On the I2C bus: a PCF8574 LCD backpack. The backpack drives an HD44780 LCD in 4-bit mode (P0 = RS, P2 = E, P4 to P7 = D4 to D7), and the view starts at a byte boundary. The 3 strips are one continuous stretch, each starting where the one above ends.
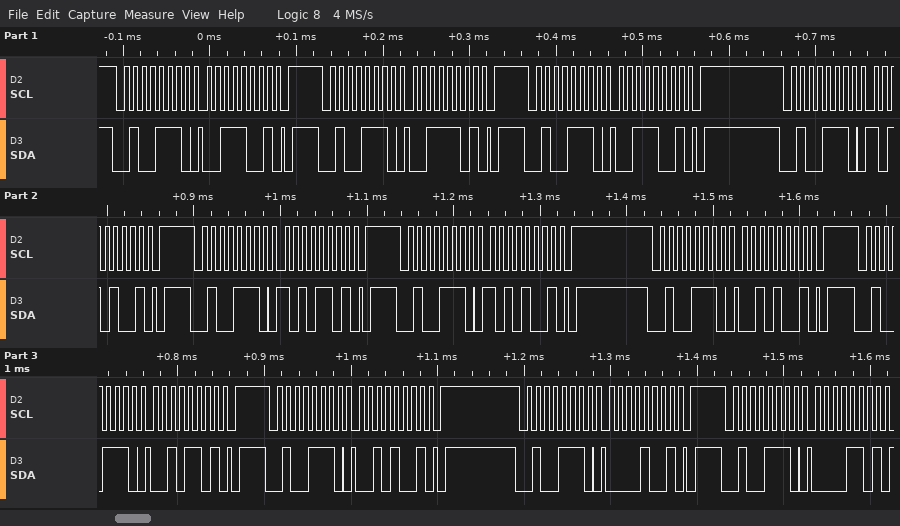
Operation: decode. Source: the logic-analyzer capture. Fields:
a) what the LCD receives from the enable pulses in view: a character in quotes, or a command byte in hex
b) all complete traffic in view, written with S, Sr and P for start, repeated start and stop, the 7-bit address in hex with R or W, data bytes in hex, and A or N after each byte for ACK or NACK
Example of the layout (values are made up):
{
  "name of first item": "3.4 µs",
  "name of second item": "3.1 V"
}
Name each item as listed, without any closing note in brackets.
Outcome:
{
  "what the LCD receives from the enable pulses in view: a character in quotes, or a command byte in hex": "':'",
  "all complete traffic in view, written with S, Sr and P for start, repeated start and stop, the 7-bit address in hex with R or W, data bytes in hex, and A or N after each byte for ACK or NACK": "S 27W A 39 A P S 27W A 3D A P S 27W A 39 A P S 27W A A9 A P S 27W A AD A P S 27W A A9 A P S 27W A 29 A P S 27W A 2D A P S 27W A 29 A P S 27W A 09 A P S 27W A 0D A"
}
